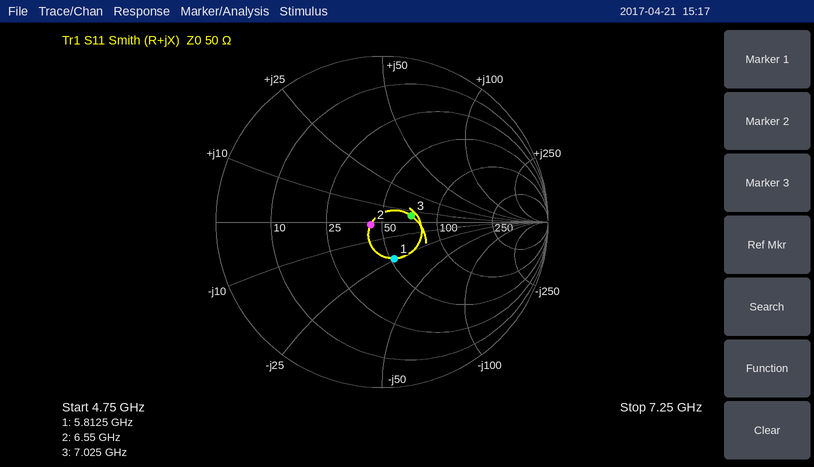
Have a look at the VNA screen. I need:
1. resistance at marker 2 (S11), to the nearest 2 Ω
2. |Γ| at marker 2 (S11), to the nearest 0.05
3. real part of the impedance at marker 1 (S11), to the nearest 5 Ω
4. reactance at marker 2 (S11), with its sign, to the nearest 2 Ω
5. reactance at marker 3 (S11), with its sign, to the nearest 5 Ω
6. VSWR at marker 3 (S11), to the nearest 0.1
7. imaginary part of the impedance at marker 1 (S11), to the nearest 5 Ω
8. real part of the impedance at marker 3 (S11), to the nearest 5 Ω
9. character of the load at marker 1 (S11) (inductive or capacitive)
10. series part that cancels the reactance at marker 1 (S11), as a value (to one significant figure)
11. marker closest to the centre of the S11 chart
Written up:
44 Ω
0.05
50 Ω
-2 Ω
+5 Ω
1.4
-25 Ω
70 Ω
capacitive
700 pH
marker 2
